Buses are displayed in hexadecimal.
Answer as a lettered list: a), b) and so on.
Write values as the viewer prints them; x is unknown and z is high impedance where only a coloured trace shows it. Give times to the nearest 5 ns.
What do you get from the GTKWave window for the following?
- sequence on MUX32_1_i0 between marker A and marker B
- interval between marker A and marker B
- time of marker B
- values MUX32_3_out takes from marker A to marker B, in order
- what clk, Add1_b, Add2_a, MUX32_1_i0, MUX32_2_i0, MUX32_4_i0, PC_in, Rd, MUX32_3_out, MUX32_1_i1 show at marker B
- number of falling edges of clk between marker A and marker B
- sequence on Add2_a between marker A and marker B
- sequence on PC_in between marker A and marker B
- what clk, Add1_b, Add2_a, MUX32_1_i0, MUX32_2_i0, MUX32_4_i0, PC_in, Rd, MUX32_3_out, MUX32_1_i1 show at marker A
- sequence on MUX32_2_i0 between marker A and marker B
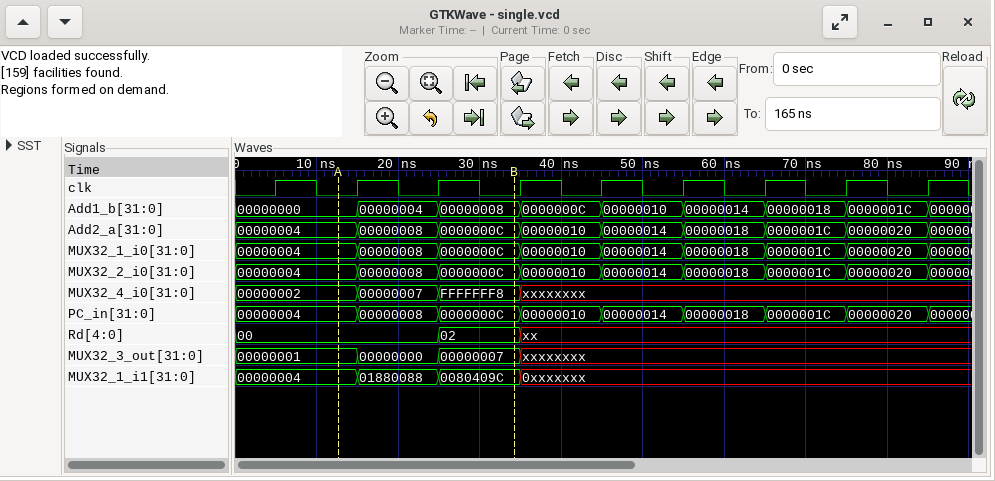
a) 00000004, 00000008, 0000000C
b) 20 ns
c) 35 ns
d) 00000001, 00000000, 00000007
e) clk=0, Add1_b=00000008, Add2_a=0000000C, MUX32_1_i0=0000000C, MUX32_2_i0=0000000C, MUX32_4_i0=FFFFFFF8, PC_in=0000000C, Rd=02, MUX32_3_out=00000007, MUX32_1_i1=0080409C
f) 2
g) 00000004, 00000008, 0000000C
h) 00000004, 00000008, 0000000C
i) clk=0, Add1_b=00000000, Add2_a=00000004, MUX32_1_i0=00000004, MUX32_2_i0=00000004, MUX32_4_i0=00000002, PC_in=00000004, Rd=00, MUX32_3_out=00000001, MUX32_1_i1=00000004
j) 00000004, 00000008, 0000000C
